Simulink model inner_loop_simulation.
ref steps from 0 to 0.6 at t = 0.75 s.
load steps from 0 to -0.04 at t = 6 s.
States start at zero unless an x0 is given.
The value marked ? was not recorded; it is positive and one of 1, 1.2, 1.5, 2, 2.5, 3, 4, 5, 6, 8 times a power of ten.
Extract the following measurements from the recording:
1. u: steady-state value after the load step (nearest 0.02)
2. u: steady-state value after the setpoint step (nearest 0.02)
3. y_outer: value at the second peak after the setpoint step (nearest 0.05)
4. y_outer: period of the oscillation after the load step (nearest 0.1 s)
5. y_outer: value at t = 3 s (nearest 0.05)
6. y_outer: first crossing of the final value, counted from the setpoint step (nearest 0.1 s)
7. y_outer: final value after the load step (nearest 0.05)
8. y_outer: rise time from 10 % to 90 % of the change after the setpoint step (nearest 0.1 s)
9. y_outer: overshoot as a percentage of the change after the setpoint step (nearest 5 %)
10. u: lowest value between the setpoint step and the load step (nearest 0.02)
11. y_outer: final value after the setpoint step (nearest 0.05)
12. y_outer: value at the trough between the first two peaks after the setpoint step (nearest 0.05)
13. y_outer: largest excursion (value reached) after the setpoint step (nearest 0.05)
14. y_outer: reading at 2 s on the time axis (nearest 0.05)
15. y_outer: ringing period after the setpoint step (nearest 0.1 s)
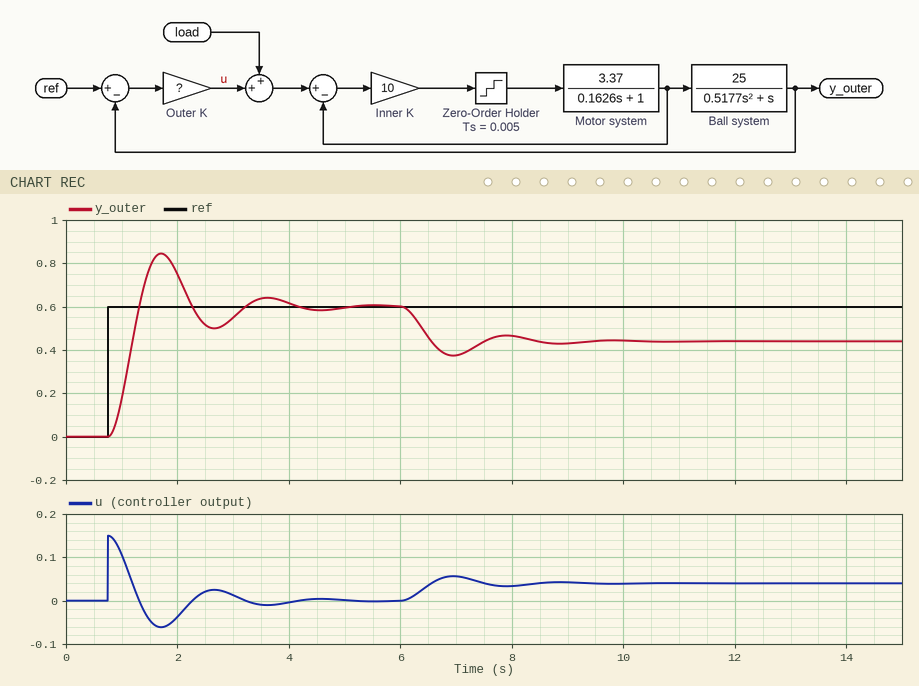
0.04
0.00
0.65
1.9 s
0.55
0.6 s
0.45
0.4 s
40 %
-0.06
0.60
0.50
0.85
0.75
1.9 s
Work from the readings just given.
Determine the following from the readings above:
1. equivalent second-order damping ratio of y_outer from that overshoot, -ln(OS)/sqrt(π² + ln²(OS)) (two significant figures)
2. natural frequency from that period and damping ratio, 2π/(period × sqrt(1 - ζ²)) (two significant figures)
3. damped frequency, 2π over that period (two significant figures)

0.28
3.4 rad/s
3.3 rad/s
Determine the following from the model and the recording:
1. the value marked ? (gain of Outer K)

0.25
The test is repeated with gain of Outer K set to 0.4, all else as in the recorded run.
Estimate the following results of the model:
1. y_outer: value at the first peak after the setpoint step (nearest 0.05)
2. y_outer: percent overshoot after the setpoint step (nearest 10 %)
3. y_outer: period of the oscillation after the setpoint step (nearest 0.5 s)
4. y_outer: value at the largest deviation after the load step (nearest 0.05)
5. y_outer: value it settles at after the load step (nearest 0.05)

0.90
50 %
1.5 s
0.45
0.50
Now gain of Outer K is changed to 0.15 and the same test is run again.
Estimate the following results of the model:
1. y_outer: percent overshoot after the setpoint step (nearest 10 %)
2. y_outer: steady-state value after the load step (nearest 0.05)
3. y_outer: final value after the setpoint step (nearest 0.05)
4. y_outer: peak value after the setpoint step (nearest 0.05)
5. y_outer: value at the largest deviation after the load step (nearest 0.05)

30 %
0.35
0.60
0.80
0.25
